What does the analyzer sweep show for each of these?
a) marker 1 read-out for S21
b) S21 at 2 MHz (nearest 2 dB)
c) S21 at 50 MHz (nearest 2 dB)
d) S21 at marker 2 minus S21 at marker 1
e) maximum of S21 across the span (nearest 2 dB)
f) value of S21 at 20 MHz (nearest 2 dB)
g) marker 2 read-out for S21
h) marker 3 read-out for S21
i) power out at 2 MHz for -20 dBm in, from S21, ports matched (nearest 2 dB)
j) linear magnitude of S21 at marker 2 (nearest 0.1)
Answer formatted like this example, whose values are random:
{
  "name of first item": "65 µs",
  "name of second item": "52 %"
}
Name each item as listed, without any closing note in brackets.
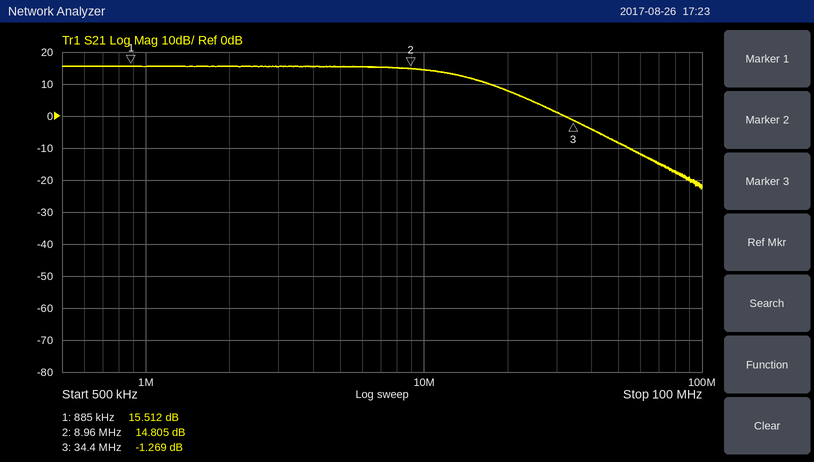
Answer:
{
  "marker 1 read-out for S21": "15.512 dB",
  "S21 at 2 MHz": "16 dB",
  "S21 at 50 MHz": "-8 dB",
  "S21 at marker 2 minus S21 at marker 1": "-0.707 dB",
  "maximum of S21 across the span": "16 dB",
  "value of S21 at 20 MHz": "8 dB",
  "marker 2 read-out for S21": "14.805 dB",
  "marker 3 read-out for S21": "-1.269 dB",
  "power out at 2 MHz for -20 dBm in, from S21, ports matched": "-4 dBm",
  "linear magnitude of S21 at marker 2": "5.5"
}
